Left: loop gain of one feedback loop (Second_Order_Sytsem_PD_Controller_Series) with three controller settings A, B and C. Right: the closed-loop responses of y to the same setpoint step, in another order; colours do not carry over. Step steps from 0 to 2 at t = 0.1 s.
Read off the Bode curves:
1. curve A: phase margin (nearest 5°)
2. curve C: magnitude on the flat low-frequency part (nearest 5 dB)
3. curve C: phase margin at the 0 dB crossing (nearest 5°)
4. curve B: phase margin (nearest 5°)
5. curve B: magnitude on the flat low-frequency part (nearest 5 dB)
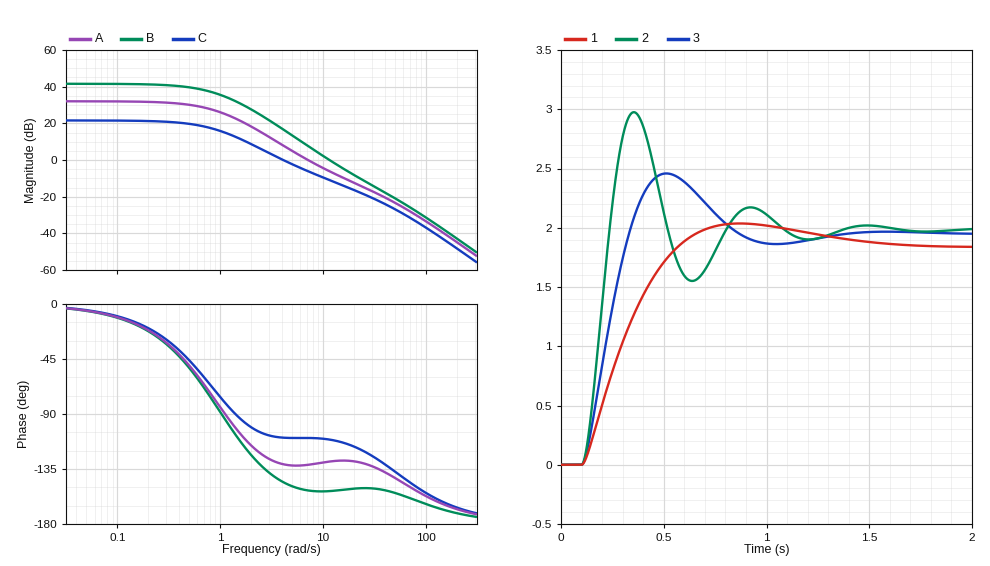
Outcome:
50°
20 dB
70°
25°
40 dB
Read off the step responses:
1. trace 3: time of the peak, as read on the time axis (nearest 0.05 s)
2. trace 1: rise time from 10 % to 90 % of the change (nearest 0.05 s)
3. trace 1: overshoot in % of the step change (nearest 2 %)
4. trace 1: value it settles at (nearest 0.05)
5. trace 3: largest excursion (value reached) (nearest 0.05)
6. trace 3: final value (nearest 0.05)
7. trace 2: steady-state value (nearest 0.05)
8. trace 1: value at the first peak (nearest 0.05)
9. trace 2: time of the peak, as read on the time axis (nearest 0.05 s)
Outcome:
0.50 s
0.35 s
10 %
1.85
2.45
1.95
2.00
2.05
0.35 s
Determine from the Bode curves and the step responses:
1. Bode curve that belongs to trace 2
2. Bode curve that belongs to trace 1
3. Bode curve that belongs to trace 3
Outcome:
B
C
A
